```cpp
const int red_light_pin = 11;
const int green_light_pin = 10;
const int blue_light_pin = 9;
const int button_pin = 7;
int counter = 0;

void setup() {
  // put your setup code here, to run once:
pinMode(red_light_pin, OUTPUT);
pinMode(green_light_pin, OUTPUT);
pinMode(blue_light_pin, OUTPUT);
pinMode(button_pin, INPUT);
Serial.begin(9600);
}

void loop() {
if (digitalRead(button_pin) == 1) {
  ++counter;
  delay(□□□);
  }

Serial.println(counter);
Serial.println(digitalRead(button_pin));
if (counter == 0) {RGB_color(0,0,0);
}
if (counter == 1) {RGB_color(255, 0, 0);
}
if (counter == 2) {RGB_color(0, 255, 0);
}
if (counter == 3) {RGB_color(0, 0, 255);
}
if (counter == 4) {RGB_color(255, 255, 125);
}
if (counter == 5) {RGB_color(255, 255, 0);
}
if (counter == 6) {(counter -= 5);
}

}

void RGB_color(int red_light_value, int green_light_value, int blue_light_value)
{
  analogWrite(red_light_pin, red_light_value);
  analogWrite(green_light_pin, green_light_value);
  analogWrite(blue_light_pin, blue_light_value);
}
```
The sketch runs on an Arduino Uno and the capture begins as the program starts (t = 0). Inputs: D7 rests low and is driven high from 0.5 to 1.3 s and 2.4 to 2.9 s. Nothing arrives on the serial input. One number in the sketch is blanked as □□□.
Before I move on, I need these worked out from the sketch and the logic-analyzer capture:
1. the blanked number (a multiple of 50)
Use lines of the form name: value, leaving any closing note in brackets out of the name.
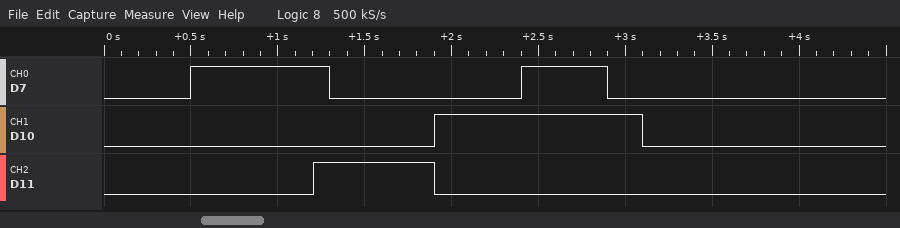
the blanked number: 700
